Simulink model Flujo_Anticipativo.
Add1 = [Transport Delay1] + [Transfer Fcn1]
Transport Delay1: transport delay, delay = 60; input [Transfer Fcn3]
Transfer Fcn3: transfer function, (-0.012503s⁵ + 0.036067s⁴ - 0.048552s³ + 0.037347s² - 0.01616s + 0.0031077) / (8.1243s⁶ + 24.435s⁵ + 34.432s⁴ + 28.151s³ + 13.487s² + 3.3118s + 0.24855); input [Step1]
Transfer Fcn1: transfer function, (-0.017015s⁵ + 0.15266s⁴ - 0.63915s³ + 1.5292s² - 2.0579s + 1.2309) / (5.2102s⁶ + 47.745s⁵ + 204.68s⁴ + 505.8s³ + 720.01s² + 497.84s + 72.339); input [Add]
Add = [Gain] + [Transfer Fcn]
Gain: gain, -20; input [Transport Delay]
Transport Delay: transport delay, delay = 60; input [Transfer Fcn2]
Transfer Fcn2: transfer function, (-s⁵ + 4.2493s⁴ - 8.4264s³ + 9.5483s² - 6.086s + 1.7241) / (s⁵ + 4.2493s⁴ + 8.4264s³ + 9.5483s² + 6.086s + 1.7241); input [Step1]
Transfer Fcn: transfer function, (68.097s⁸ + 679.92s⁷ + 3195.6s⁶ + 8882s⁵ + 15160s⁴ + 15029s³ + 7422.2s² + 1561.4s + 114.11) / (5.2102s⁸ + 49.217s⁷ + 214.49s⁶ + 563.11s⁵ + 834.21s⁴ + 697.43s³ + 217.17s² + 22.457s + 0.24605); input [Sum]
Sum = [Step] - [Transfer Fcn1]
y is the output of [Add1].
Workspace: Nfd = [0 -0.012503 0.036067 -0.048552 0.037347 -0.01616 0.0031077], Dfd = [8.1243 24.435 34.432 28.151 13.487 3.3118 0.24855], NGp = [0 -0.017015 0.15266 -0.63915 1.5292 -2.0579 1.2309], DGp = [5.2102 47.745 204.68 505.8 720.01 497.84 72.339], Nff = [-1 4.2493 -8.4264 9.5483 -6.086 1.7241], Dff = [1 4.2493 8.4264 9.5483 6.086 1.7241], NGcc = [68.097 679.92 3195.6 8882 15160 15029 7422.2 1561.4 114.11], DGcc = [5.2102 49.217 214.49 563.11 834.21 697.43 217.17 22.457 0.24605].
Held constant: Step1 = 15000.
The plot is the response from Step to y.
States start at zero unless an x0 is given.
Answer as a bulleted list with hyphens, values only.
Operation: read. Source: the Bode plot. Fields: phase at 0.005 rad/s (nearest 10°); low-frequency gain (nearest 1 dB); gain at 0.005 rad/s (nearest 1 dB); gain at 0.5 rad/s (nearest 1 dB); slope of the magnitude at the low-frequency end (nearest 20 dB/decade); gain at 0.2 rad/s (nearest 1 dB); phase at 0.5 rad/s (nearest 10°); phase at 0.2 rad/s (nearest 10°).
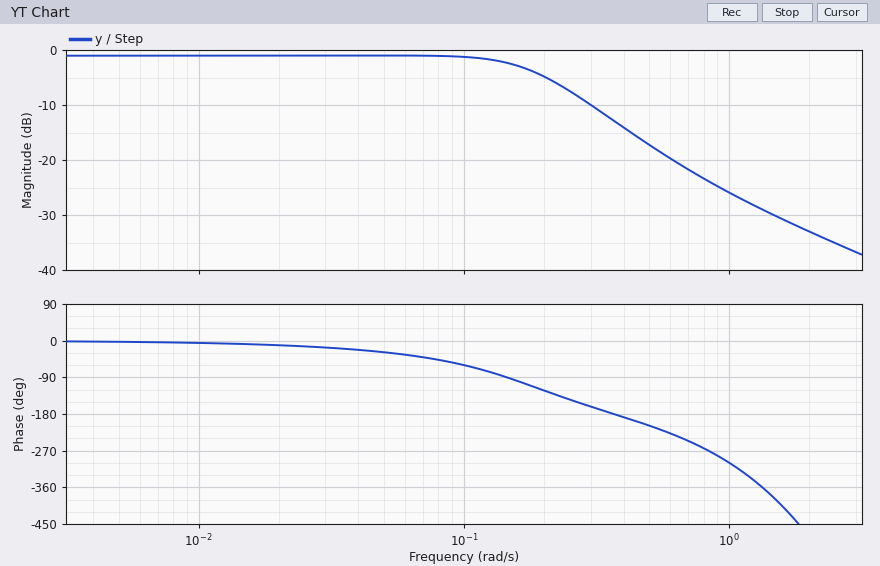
- 0°
- -1 dB
- -1 dB
- -17 dB
- 0 dB/decade
- -5 dB
- -210°
- -120°
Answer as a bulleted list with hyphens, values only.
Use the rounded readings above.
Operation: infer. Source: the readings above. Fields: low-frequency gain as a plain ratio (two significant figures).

- 0.89
